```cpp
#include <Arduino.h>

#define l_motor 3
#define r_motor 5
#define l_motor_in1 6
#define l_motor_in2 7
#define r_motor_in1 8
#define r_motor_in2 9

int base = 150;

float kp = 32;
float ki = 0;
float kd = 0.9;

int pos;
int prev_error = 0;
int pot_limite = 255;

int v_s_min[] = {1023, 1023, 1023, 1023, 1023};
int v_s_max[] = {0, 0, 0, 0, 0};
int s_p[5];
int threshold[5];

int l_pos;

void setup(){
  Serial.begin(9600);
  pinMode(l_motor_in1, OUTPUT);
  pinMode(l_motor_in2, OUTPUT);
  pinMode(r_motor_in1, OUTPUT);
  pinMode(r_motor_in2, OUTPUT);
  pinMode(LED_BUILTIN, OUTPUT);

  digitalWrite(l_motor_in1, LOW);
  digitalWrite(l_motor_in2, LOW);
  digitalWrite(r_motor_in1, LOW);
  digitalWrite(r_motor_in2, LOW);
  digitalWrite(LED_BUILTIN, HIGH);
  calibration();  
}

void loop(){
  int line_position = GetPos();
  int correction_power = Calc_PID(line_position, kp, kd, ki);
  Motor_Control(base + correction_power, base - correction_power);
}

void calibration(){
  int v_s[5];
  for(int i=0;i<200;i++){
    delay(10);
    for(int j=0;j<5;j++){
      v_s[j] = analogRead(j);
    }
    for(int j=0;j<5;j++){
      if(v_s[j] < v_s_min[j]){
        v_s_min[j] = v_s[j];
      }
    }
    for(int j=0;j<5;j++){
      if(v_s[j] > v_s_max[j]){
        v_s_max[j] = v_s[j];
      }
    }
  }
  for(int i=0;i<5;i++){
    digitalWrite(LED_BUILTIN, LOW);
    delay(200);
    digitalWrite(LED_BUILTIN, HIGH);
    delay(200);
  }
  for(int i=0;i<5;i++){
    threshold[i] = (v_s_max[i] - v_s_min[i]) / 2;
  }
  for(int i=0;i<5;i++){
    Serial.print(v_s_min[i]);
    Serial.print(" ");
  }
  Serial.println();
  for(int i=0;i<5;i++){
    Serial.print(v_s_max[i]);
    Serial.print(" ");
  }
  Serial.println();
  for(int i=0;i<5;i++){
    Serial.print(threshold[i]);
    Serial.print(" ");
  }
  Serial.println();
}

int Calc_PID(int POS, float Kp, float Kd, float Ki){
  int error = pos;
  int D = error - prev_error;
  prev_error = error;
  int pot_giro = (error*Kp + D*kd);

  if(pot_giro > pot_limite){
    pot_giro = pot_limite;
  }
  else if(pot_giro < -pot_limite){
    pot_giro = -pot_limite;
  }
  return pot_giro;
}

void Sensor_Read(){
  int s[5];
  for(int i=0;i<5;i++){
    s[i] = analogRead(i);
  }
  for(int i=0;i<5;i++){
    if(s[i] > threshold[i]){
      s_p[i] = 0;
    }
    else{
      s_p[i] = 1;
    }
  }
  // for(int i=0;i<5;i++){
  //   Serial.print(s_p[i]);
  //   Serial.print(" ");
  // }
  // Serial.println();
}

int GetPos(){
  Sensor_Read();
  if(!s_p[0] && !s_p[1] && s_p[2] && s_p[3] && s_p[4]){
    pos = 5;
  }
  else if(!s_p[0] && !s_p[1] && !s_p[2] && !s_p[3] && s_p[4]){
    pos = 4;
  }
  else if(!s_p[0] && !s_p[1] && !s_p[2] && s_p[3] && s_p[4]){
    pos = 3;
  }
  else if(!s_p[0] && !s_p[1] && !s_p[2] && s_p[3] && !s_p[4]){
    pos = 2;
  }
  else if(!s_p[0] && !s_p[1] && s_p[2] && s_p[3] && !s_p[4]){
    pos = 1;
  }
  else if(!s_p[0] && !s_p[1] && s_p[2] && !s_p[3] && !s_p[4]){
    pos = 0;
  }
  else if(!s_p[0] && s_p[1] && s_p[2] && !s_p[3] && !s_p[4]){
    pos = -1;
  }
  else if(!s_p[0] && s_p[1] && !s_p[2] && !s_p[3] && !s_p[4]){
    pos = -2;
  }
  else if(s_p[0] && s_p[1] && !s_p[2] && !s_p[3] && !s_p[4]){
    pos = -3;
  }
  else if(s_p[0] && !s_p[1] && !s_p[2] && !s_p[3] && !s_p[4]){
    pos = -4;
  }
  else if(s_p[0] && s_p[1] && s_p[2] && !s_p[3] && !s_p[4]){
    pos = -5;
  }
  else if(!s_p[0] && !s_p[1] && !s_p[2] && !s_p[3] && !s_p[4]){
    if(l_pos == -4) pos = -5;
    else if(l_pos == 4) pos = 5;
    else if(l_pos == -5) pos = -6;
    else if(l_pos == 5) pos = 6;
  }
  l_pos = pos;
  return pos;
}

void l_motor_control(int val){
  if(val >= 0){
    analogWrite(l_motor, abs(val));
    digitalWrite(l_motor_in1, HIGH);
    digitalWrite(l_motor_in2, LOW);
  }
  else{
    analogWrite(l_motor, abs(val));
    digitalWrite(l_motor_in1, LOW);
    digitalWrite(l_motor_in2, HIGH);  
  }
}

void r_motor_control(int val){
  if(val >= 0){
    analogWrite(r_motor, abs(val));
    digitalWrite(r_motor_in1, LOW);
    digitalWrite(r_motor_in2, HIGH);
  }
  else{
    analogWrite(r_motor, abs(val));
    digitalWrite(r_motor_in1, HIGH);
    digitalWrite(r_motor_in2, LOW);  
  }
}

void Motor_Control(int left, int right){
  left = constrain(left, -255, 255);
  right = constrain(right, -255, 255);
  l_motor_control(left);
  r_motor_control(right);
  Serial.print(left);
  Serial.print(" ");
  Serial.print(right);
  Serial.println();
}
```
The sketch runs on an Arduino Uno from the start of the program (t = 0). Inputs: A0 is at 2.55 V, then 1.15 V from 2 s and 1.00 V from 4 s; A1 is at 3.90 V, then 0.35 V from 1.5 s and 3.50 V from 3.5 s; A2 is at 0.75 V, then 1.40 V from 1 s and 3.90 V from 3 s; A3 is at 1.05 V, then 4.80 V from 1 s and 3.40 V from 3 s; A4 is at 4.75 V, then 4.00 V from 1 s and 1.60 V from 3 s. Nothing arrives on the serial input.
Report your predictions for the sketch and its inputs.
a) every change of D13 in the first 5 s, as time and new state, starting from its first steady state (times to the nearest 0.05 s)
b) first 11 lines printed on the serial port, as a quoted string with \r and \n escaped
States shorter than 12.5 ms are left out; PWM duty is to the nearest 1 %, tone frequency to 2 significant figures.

0 s high; 2.1 s low; 2.3 s high; 2.5 s low; 2.7 s high; 2.9 s low; 3.1 s high; 3.3 s low; 3.5 s high; 3.7 s low; 3.9 s high
"235 71 153 215 819 \r\n522 798 286 983 972 \r\n143 363 66 384 76 \r\n150 150\r\n150 150\r\n150 150\r\n150 150\r\n150 150\r\n150 150\r\n150 150\r\n150 150\r\n"
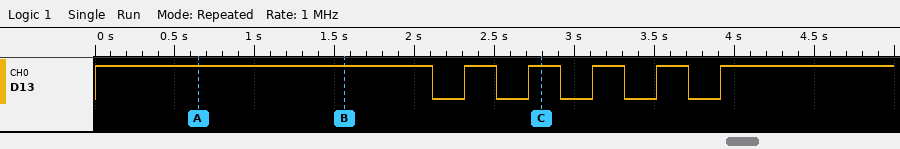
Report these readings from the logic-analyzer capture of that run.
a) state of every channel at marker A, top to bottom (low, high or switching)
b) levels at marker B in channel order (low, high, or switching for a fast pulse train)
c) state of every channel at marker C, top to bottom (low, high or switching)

D13 high
D13 high
D13 high
